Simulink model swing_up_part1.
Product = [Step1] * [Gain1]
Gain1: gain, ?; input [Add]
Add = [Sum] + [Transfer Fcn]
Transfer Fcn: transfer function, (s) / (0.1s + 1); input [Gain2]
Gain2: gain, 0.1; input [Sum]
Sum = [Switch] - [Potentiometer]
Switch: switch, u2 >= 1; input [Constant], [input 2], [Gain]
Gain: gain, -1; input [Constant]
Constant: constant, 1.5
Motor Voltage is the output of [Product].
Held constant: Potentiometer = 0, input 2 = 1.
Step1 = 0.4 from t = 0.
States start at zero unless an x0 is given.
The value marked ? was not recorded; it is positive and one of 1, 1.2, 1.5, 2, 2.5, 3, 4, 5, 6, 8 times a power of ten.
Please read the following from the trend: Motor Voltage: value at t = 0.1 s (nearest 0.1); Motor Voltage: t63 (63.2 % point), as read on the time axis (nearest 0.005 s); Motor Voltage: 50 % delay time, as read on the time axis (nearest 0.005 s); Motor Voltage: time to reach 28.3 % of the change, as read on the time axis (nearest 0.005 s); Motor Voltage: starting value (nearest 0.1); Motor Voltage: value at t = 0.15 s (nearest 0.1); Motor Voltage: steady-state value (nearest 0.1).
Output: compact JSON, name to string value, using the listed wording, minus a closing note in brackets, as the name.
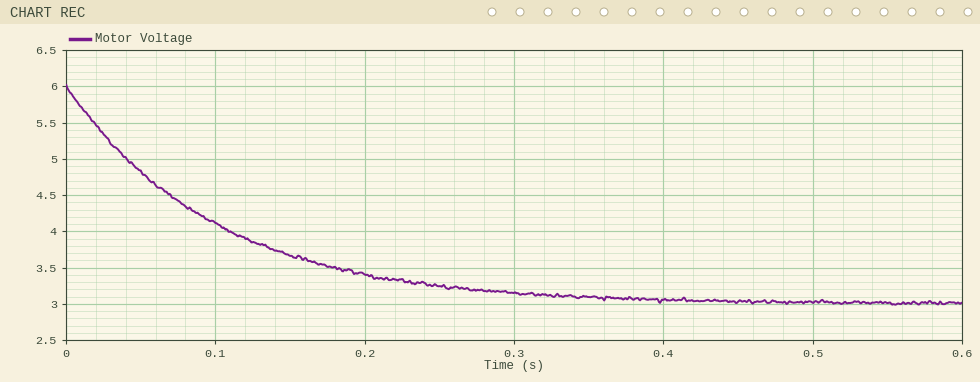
{"Motor Voltage: value at t = 0.1 s": "4.1", "Motor Voltage: t63 (63.2 % point), as read on the time axis": "0.100 s", "Motor Voltage: 50 % delay time, as read on the time axis": "0.070 s", "Motor Voltage: time to reach 28.3 % of the change, as read on the time axis": "0.035 s", "Motor Voltage: starting value": "6.0", "Motor Voltage: value at t = 0.15 s": "3.7", "Motor Voltage: steady-state value": "3.0"}
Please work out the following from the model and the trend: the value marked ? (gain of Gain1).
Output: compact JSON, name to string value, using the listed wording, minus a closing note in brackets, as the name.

{"the value marked ?": "5"}
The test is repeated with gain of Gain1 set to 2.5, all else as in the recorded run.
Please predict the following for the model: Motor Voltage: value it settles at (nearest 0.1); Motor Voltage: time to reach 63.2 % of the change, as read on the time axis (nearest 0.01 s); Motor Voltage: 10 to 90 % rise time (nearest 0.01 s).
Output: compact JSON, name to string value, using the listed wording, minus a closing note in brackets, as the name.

{"Motor Voltage: value it settles at": "1.5", "Motor Voltage: time to reach 63.2 % of the change, as read on the time axis": "0.10 s", "Motor Voltage: 10 to 90 % rise time": "0.22 s"}
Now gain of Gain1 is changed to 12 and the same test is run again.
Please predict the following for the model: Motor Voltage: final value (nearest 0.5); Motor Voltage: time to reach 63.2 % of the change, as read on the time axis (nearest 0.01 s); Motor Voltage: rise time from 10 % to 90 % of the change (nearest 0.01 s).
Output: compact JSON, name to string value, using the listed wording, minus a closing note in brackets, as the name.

{"Motor Voltage: final value": "7.0", "Motor Voltage: time to reach 63.2 % of the change, as read on the time axis": "0.10 s", "Motor Voltage: rise time from 10 % to 90 % of the change": "0.22 s"}
